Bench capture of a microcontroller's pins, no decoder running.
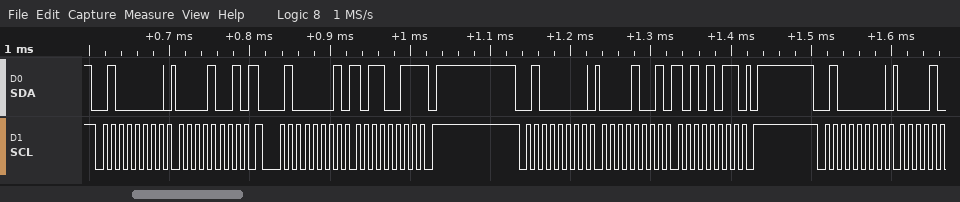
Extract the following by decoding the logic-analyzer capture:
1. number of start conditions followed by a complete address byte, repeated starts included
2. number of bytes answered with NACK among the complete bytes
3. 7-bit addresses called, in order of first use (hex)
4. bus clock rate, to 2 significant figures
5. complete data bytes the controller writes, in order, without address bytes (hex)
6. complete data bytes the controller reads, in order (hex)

4
1
0x20
100 kHz
09 09 AB
B3
